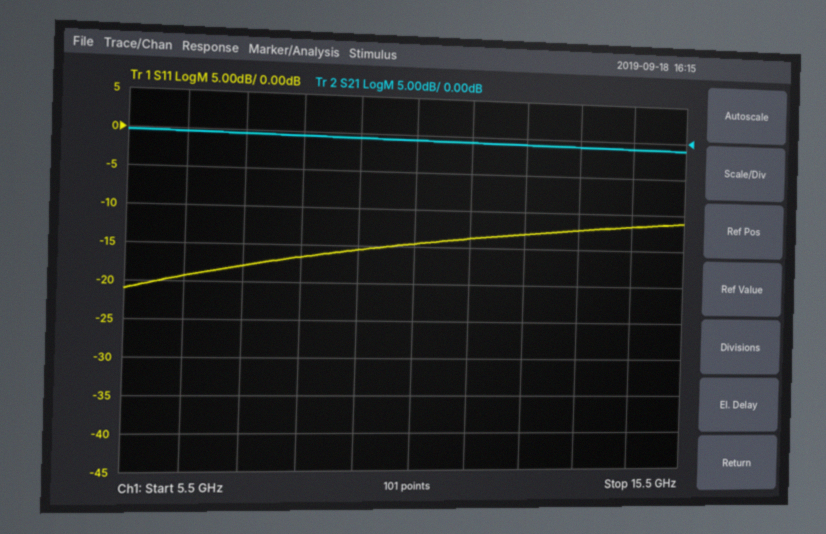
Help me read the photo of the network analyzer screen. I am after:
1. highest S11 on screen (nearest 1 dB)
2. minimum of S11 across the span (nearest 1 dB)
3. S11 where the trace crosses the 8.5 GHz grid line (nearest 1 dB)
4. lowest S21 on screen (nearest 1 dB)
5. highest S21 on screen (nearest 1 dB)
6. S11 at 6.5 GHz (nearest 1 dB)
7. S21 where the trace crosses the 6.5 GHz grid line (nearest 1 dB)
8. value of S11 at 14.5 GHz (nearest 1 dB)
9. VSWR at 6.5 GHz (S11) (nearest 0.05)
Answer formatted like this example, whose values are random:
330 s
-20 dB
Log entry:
-11 dB
-21 dB
-17 dB
-1 dB
0 dB
-19 dB
0 dB
-12 dB
1.25
